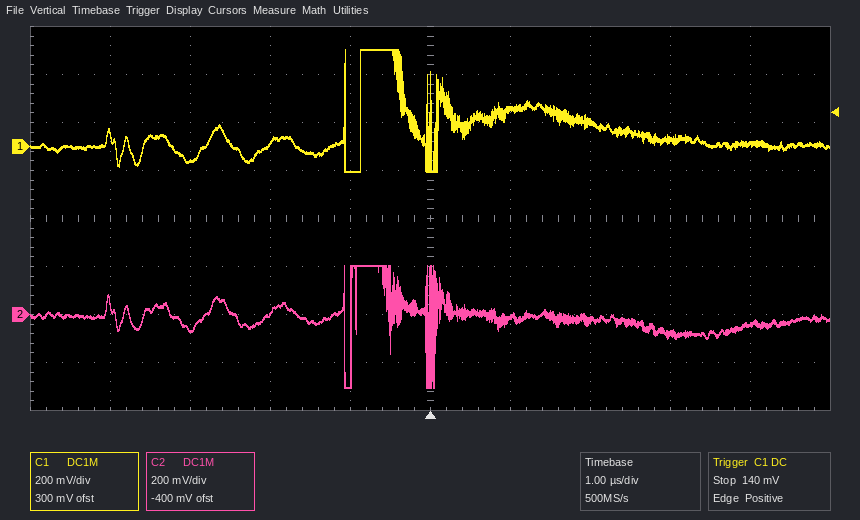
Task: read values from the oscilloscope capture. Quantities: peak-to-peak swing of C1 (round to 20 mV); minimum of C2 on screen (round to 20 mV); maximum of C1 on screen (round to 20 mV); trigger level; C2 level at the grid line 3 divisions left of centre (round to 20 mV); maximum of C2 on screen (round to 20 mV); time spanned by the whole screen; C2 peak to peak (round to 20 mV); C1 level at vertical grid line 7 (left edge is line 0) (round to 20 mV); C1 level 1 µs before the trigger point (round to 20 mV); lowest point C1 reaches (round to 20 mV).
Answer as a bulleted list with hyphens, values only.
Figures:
- 500 mV
- -300 mV
- 400 mV
- 140 mV
- -60 mV
- 200 mV
- 10 µs
- 500 mV
- 100 mV
- -100 mV
- -100 mV
